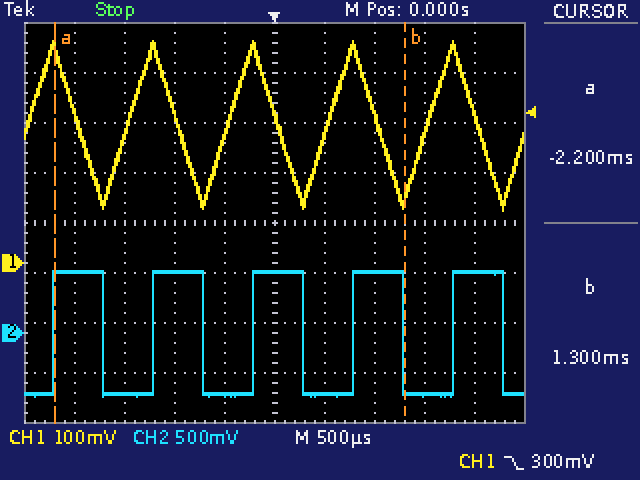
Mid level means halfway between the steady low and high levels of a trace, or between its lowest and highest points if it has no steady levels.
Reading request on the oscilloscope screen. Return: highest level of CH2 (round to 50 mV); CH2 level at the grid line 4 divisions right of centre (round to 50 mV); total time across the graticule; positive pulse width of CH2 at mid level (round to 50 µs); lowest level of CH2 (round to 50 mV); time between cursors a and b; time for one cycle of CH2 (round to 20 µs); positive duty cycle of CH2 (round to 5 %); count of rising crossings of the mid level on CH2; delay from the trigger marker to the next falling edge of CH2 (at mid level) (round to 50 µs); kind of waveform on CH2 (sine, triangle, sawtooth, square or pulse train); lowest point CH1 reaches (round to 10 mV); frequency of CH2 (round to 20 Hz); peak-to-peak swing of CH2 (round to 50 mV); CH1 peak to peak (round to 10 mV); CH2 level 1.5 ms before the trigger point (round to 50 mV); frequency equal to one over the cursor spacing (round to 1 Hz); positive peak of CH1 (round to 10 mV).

600 mV
600 mV
5 ms
500 µs
-650 mV
3.50 ms
1.00 ms
50 %
5
300 µs
square
100 mV
1.00 kHz
1.25 V
340 mV
-600 mV
286 Hz
440 mV
